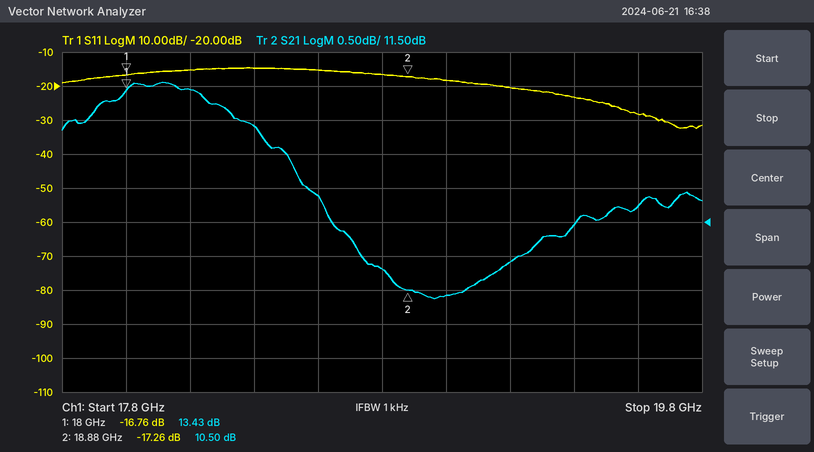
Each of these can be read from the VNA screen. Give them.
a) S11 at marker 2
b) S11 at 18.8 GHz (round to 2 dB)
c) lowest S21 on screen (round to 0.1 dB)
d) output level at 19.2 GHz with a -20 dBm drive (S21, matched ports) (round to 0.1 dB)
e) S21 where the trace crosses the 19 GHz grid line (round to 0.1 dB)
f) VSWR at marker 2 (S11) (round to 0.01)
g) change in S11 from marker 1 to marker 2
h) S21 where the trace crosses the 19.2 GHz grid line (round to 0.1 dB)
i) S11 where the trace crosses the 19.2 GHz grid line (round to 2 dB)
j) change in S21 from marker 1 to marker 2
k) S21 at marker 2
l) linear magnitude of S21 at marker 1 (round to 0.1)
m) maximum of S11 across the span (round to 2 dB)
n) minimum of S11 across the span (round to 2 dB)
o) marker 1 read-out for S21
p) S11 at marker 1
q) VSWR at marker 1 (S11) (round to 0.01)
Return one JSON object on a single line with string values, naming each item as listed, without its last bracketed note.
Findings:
{"S11 at marker 2": "-17.26 dB", "S11 at 18.8 GHz": "-16 dB", "lowest S21 on screen": "10.4 dB", "output level at 19.2 GHz with a -20 dBm drive (S21, matched ports)": "-9.1 dBm", "S21 where the trace crosses the 19 GHz grid line": "10.4 dB", "VSWR at marker 2 (S11)": "1.32", "change in S11 from marker 1 to marker 2": "-0.50 dB", "S21 where the trace crosses the 19.2 GHz grid line": "10.9 dB", "S11 where the trace crosses the 19.2 GHz grid line": "-20 dB", "change in S21 from marker 1 to marker 2": "-2.93 dB", "S21 at marker 2": "10.50 dB", "linear magnitude of S21 at marker 1": "4.7", "maximum of S11 across the span": "-14 dB", "minimum of S11 across the span": "-32 dB", "marker 1 read-out for S21": "13.43 dB", "S11 at marker 1": "-16.76 dB", "VSWR at marker 1 (S11)": "1.34"}
